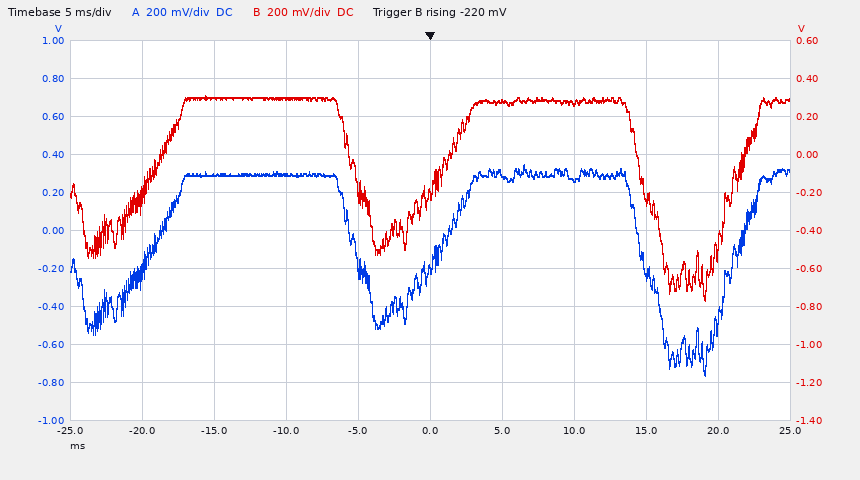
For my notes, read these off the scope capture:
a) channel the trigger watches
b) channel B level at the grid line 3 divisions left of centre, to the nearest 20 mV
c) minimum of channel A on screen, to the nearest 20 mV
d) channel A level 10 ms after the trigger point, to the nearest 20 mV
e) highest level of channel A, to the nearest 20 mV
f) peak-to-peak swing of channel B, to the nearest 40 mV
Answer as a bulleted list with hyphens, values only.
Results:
- channel B
- 300 mV
- -760 mV
- 260 mV
- 340 mV
- 1.08 V
